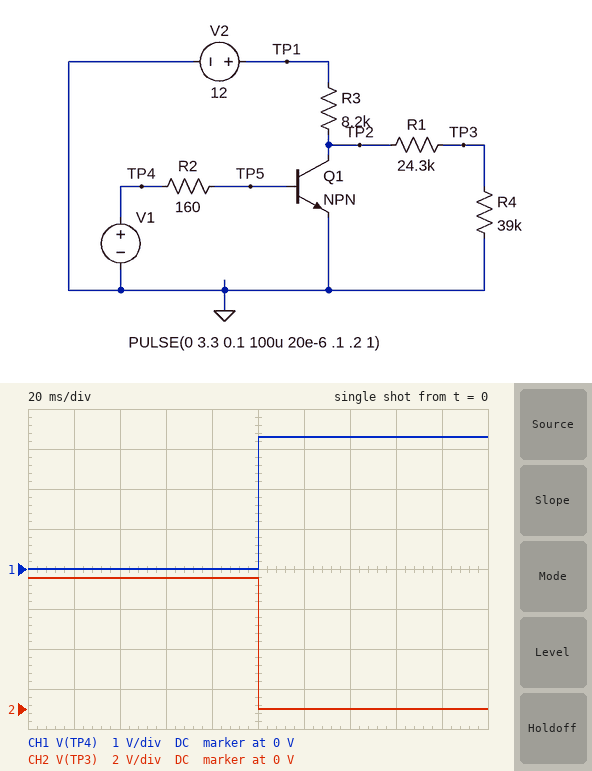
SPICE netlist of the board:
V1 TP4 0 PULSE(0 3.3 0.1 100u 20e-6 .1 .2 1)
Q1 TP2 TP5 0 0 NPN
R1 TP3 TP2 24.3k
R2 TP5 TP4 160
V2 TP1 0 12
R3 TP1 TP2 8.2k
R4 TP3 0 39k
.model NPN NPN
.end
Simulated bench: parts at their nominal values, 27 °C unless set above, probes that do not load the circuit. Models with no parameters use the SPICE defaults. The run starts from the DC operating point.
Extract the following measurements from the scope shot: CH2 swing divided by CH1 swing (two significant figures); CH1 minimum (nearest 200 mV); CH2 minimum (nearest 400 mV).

2.0
0 V
0 V
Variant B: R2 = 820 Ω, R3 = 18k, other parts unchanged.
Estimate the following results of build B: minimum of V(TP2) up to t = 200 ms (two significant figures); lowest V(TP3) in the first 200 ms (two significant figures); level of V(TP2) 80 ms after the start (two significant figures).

21 mV
13 mV
9.3 V
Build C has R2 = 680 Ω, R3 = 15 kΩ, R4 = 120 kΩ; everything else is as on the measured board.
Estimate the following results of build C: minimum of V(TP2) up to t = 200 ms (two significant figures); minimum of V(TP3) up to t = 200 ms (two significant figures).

21 mV
17 mV
